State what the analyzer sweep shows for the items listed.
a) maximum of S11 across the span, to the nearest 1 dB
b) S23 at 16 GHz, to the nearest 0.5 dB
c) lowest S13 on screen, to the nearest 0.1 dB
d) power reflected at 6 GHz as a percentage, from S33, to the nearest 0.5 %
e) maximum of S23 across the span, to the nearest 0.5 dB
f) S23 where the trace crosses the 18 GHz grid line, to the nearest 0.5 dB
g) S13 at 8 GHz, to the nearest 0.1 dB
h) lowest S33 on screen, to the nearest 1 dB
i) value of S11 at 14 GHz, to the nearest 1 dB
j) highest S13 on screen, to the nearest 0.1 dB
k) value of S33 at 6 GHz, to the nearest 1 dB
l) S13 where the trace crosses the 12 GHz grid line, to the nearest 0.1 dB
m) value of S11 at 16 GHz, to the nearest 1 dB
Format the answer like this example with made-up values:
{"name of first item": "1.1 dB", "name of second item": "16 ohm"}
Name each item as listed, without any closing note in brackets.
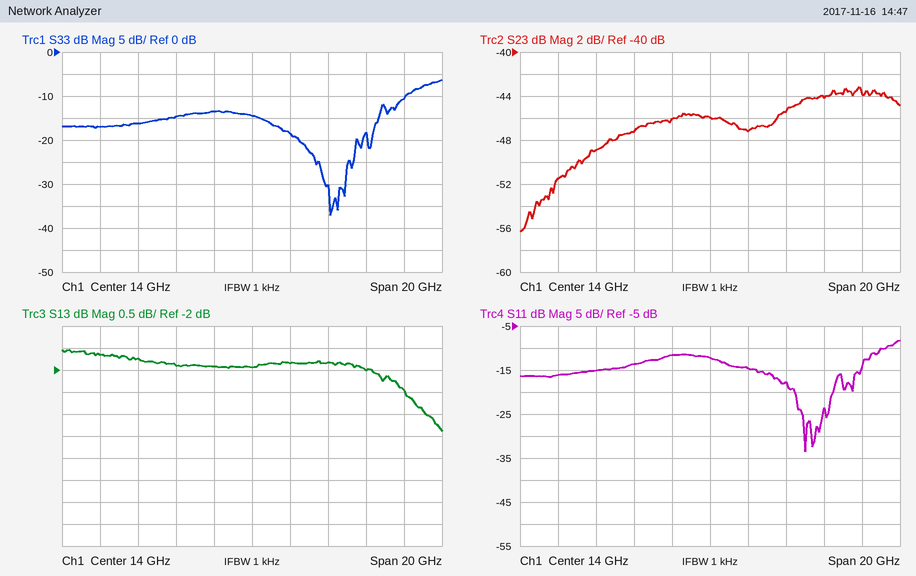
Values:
{"maximum of S11 across the span, to the nearest 1 dB": "-8 dB", "S23 at 16 GHz, to the nearest 0.5 dB": "-47.0 dB", "lowest S13 on screen, to the nearest 0.1 dB": "-3.4 dB", "power reflected at 6 GHz as a percentage, from S33, to the nearest 0.5 %": "2.0 %", "maximum of S23 across the span, to the nearest 0.5 dB": "-43.0 dB", "S23 where the trace crosses the 18 GHz grid line, to the nearest 0.5 dB": "-45.5 dB", "S13 at 8 GHz, to the nearest 0.1 dB": "-1.7 dB", "lowest S33 on screen, to the nearest 1 dB": "-37 dB", "value of S11 at 14 GHz, to the nearest 1 dB": "-12 dB", "highest S13 on screen, to the nearest 0.1 dB": "-1.5 dB", "value of S33 at 6 GHz, to the nearest 1 dB": "-17 dB", "S13 where the trace crosses the 12 GHz grid line, to the nearest 0.1 dB": "-1.9 dB", "value of S11 at 16 GHz, to the nearest 1 dB": "-15 dB"}
